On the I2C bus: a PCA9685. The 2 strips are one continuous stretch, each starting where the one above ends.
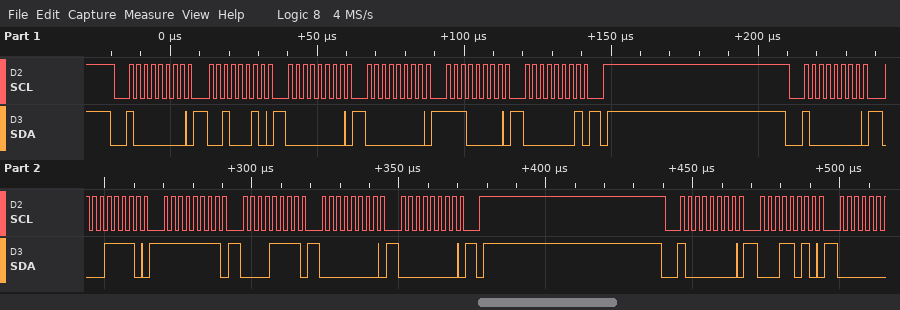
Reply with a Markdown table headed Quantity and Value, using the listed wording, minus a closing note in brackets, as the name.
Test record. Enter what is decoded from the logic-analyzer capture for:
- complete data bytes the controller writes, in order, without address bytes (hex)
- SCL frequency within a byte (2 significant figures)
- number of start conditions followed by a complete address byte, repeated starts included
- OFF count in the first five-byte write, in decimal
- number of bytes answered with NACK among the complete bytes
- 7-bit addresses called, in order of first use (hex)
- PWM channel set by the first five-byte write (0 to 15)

| Quantity | Value |
|---|---|
| complete data bytes the controller writes, in order, without address bytes | 22 00 00 E0 01 1E FF 0F 00 00 1A |
| SCL frequency within a byte | 400 kHz |
| number of start conditions followed by a complete address byte, repeated starts included | 3 |
| OFF count in the first five-byte write, in decimal | 480 |
| number of bytes answered with NACK among the complete bytes | 0 |
| 7-bit addresses called, in order of first use | 0x40 |
| PWM channel set by the first five-byte write | 7 |
